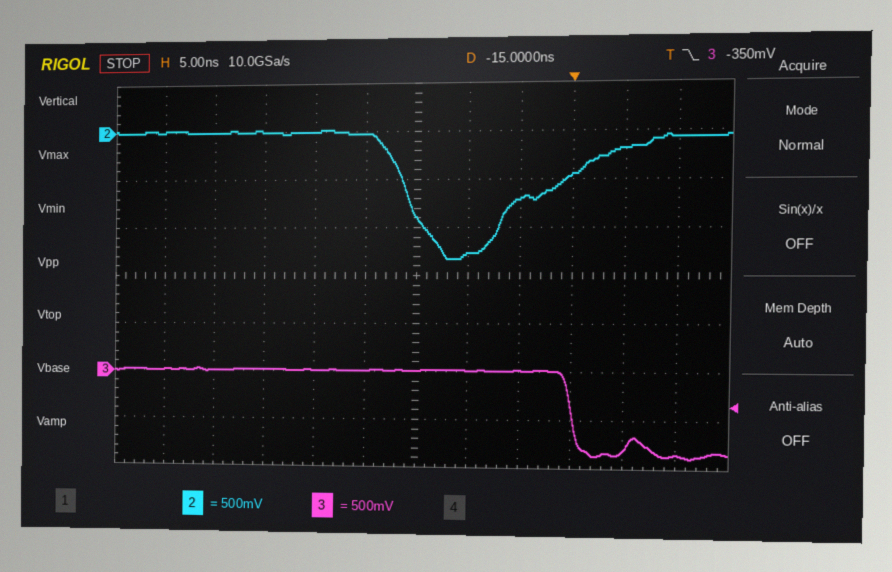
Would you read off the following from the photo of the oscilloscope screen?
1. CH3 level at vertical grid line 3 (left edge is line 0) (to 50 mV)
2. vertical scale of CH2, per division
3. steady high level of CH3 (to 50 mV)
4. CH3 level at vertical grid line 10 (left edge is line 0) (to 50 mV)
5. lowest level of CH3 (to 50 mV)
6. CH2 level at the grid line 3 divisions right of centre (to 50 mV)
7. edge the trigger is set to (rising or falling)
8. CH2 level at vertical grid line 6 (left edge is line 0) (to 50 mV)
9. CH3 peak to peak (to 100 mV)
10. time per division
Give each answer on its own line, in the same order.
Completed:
0 mV
500 mV
0 mV
-800 mV
-900 mV
-450 mV
falling
-900 mV
900 mV
5 ns
